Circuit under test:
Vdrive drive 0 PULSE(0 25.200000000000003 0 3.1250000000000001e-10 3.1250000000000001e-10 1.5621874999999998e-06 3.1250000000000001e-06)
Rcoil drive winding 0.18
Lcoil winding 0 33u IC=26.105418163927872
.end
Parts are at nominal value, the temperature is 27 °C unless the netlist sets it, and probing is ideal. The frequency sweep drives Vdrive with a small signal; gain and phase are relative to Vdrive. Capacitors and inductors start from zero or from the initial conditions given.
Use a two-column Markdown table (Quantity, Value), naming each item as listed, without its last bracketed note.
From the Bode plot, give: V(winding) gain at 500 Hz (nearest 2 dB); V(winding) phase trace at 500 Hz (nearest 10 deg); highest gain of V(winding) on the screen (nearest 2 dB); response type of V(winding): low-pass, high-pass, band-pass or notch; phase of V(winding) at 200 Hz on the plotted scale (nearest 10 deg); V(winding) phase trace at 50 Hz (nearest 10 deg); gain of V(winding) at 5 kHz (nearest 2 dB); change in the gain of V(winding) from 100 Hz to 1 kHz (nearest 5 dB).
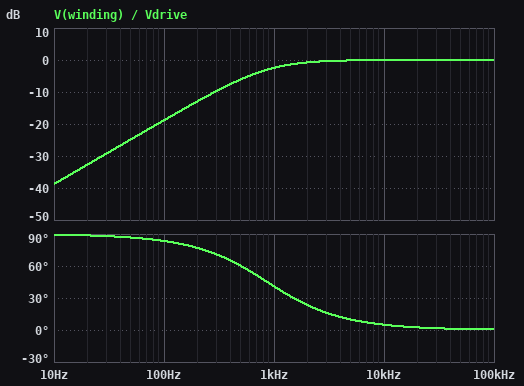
| Quantity | Value |
|---|---|
| V(winding) gain at 500 Hz | -6 dB |
| V(winding) phase trace at 500 Hz | 60 deg |
| highest gain of V(winding) on the screen | 0 dB |
| response type of V(winding): low-pass, high-pass, band-pass or notch | high-pass |
| phase of V(winding) at 200 Hz on the plotted scale | 80 deg |
| V(winding) phase trace at 50 Hz | 90 deg |
| gain of V(winding) at 5 kHz | 0 dB |
| change in the gain of V(winding) from 100 Hz to 1 kHz | 15 dB |
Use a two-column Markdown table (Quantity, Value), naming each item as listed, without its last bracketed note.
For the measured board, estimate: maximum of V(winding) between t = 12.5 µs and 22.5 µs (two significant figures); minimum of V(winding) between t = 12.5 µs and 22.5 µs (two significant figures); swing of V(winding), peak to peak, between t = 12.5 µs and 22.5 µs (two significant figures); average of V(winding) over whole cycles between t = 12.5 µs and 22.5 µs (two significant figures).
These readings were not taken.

| Quantity | Value |
|---|---|
| maximum of V(winding) between t = 12.5 µs and 22.5 µs | 20 V |
| minimum of V(winding) between t = 12.5 µs and 22.5 µs | -5.6 V |
| swing of V(winding), peak to peak, between t = 12.5 µs and 22.5 µs | 26 V |
| average of V(winding) over whole cycles between t = 12.5 µs and 22.5 µs | 7.1 V |
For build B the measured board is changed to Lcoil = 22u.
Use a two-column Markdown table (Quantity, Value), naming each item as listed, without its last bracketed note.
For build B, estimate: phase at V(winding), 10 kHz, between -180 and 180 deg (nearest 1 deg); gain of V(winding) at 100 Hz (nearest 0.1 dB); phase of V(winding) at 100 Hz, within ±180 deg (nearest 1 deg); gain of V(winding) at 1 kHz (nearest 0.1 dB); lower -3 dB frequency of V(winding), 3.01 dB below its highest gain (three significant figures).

| Quantity | Value |
|---|---|
| phase at V(winding), 10 kHz, between -180 and 180 deg | 7 deg |
| gain of V(winding) at 100 Hz | -22.3 dB |
| phase of V(winding) at 100 Hz, within ±180 deg | 86 deg |
| gain of V(winding) at 1 kHz | -4.3 dB |
| lower -3 dB frequency of V(winding), 3.01 dB below its highest gain | 1.30 kHz |
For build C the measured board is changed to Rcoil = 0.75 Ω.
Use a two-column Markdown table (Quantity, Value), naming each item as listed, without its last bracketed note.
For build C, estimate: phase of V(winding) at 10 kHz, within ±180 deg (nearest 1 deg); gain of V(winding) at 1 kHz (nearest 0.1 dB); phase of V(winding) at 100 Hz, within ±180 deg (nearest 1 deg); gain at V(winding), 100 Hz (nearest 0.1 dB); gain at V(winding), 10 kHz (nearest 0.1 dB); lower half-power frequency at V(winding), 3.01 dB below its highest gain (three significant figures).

| Quantity | Value |
|---|---|
| phase of V(winding) at 10 kHz, within ±180 deg | 20 deg |
| gain of V(winding) at 1 kHz | -11.5 dB |
| phase of V(winding) at 100 Hz, within ±180 deg | 88 deg |
| gain at V(winding), 100 Hz | -31.2 dB |
| gain at V(winding), 10 kHz | -0.5 dB |
| lower half-power frequency at V(winding), 3.01 dB below its highest gain | 3.62 kHz |
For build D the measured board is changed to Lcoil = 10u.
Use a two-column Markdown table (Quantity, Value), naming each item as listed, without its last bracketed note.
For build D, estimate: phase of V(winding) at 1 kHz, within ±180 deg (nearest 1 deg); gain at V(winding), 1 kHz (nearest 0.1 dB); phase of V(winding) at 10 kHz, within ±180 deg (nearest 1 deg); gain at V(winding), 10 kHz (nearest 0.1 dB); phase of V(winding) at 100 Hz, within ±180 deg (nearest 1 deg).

| Quantity | Value |
|---|---|
| phase of V(winding) at 1 kHz, within ±180 deg | 71 deg |
| gain at V(winding), 1 kHz | -9.6 dB |
| phase of V(winding) at 10 kHz, within ±180 deg | 16 deg |
| gain at V(winding), 10 kHz | -0.3 dB |
| phase of V(winding) at 100 Hz, within ±180 deg | 88 deg |
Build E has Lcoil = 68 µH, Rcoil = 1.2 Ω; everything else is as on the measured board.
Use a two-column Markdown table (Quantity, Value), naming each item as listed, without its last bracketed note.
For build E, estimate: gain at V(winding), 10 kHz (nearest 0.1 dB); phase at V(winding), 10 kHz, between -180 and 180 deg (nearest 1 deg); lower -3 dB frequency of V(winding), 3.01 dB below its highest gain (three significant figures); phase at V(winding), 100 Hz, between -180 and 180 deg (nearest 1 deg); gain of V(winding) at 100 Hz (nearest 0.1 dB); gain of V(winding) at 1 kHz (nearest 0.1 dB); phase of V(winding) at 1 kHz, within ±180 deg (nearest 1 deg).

| Quantity | Value |
|---|---|
| gain at V(winding), 10 kHz | -0.3 dB |
| phase at V(winding), 10 kHz, between -180 and 180 deg | 16 deg |
| lower -3 dB frequency of V(winding), 3.01 dB below its highest gain | 2.81 kHz |
| phase at V(winding), 100 Hz, between -180 and 180 deg | 88 deg |
| gain of V(winding) at 100 Hz | -29.0 dB |
| gain of V(winding) at 1 kHz | -9.5 dB |
| phase of V(winding) at 1 kHz, within ±180 deg | 70 deg |
